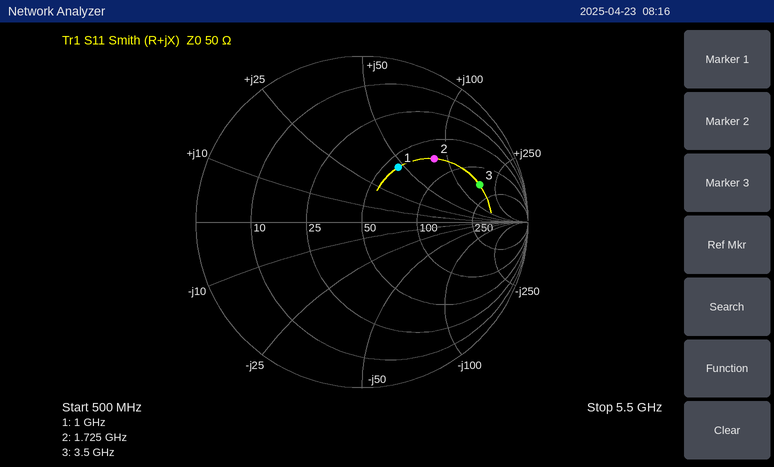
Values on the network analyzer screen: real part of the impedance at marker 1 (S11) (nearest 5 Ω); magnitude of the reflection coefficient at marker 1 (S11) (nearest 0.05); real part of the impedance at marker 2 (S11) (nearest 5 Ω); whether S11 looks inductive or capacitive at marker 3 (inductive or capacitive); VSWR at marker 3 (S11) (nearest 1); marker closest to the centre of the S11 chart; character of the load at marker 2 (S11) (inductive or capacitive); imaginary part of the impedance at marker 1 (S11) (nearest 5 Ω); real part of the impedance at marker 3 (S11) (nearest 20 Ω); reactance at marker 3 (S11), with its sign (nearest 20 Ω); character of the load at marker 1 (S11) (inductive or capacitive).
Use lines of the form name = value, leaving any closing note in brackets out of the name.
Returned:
real part of the impedance at marker 1 (S11) = 60 Ω
magnitude of the reflection coefficient at marker 1 (S11) = 0.40
real part of the impedance at marker 2 (S11) = 70 Ω
whether S11 looks inductive or capacitive at marker 3 = inductive
VSWR at marker 3 (S11) = 7
marker closest to the centre of the S11 chart = marker 1
character of the load at marker 2 (S11) = inductive
imaginary part of the impedance at marker 1 (S11) = +45 Ω
real part of the impedance at marker 3 (S11) = 160 Ω
reactance at marker 3 (S11), with its sign = +160 Ω
character of the load at marker 1 (S11) = inductive
